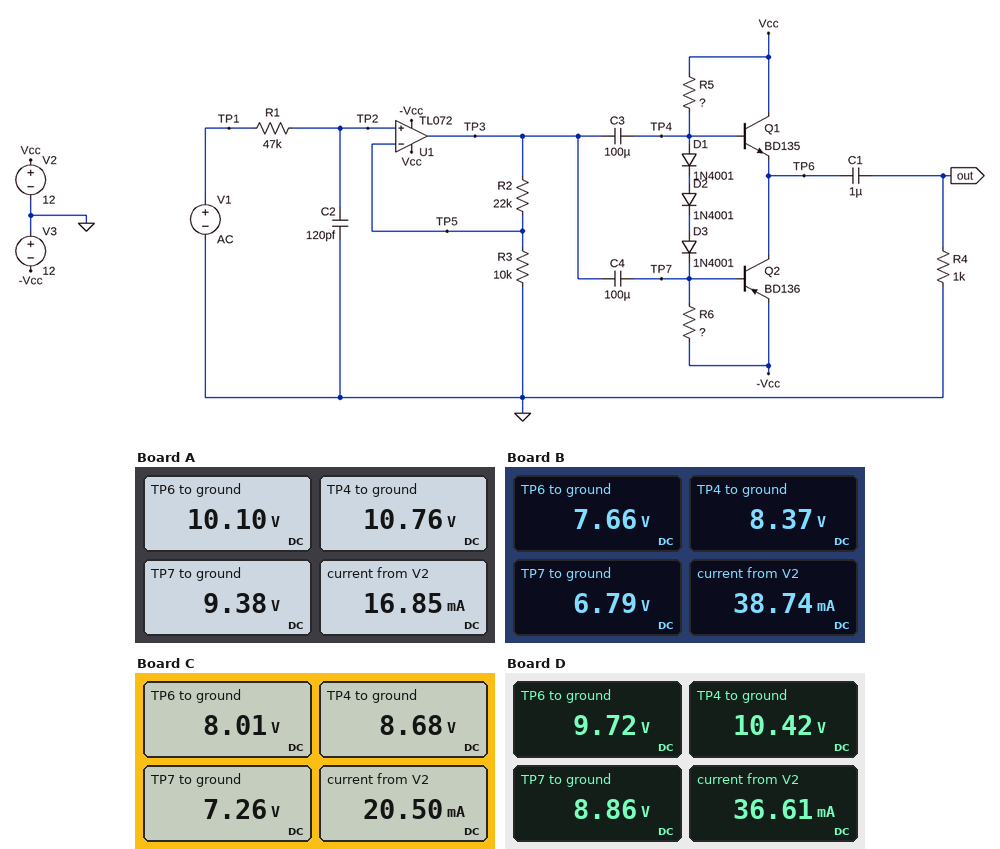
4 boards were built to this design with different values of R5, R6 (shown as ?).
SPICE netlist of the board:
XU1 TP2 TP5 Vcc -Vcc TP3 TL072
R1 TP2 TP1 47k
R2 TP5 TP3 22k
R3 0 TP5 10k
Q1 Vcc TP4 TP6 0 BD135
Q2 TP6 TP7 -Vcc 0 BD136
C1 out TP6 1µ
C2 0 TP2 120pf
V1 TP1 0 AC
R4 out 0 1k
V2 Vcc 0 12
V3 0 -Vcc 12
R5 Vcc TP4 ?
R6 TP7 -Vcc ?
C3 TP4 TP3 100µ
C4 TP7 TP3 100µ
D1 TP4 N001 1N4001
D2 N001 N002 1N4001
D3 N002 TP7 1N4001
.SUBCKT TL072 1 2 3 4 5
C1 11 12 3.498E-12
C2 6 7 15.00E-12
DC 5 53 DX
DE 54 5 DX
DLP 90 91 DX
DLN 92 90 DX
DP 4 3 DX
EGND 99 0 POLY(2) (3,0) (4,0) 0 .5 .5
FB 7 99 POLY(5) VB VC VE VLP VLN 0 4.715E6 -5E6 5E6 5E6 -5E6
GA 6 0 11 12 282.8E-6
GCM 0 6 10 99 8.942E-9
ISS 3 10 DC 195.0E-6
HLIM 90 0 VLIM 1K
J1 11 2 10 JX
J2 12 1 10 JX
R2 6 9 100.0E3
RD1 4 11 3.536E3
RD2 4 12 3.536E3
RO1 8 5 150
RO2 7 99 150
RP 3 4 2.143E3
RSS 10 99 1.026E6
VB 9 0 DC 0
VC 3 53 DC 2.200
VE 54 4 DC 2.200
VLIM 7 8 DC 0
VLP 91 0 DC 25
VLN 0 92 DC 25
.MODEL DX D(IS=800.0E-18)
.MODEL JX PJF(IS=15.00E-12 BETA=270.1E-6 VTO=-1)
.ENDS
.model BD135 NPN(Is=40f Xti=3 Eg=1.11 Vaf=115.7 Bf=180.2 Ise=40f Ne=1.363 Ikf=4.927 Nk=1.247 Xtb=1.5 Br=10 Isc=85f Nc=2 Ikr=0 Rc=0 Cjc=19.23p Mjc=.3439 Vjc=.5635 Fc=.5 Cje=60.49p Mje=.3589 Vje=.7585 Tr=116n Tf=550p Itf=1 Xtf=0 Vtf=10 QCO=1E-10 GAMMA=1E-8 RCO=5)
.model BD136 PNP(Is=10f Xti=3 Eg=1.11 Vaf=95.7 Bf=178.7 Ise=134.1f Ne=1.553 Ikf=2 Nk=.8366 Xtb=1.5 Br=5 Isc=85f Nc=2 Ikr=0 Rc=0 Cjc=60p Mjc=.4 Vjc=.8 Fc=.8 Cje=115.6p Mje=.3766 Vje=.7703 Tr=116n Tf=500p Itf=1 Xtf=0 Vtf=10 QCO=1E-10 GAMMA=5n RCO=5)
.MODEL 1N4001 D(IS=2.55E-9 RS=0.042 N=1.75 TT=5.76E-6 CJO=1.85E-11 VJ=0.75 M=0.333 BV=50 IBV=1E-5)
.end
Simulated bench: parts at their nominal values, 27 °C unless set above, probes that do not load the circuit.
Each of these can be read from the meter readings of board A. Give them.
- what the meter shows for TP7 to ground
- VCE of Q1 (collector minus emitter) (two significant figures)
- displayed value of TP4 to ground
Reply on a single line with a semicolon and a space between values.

9.38 V; 1.9 V; 10.76 V
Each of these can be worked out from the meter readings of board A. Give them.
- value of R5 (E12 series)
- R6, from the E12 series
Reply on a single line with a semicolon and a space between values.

12 kΩ; 22 kΩ
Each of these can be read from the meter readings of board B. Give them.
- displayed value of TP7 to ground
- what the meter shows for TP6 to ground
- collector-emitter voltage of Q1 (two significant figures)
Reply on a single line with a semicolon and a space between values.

6.79 V; 7.66 V; 4.3 V
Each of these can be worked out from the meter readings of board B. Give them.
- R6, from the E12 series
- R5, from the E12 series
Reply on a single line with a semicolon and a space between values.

3.9 kΩ; 8.2 kΩ
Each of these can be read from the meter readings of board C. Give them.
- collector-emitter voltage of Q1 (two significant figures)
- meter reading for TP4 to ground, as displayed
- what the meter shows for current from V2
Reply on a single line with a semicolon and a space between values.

4.0 V; 8.68 V; 20.50 mA
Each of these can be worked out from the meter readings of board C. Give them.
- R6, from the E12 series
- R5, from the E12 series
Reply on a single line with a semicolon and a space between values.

12 kΩ; 22 kΩ
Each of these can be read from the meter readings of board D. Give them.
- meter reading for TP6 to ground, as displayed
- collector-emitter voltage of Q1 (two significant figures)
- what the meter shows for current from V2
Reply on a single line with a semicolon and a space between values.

9.72 V; 2.3 V; 36.61 mA
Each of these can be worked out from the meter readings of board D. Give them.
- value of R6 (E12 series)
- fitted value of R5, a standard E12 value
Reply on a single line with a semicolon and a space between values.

4.7 kΩ; 3.9 kΩ
